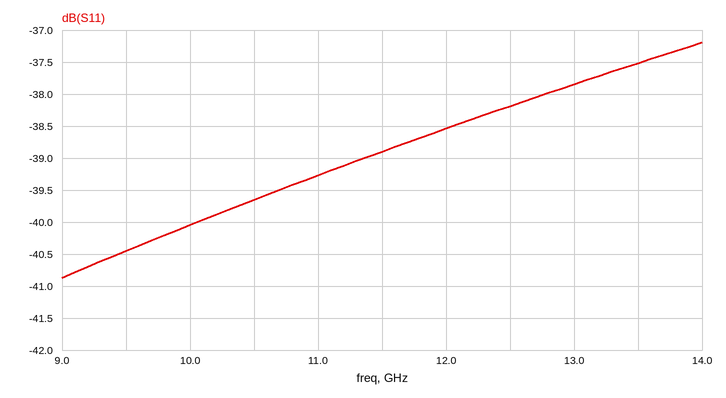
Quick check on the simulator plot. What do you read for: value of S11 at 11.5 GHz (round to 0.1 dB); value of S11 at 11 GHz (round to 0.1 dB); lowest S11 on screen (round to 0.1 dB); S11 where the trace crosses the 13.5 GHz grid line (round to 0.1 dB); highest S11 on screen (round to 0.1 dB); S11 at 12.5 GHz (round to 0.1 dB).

-38.9 dB
-39.3 dB
-40.9 dB
-37.5 dB
-37.2 dB
-38.2 dB
